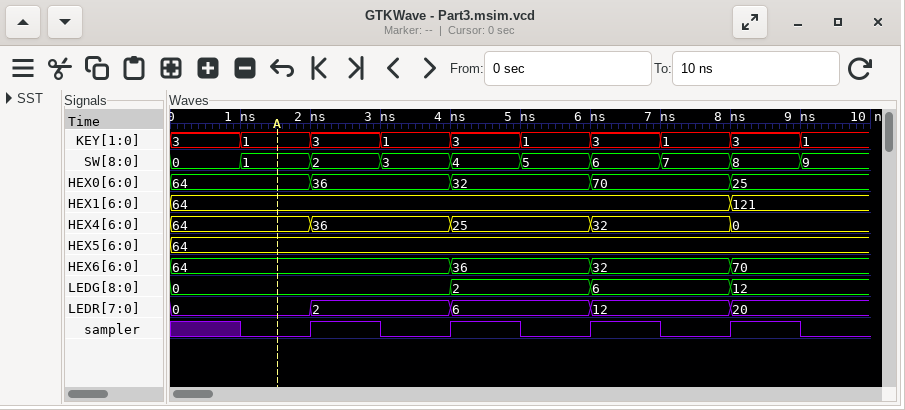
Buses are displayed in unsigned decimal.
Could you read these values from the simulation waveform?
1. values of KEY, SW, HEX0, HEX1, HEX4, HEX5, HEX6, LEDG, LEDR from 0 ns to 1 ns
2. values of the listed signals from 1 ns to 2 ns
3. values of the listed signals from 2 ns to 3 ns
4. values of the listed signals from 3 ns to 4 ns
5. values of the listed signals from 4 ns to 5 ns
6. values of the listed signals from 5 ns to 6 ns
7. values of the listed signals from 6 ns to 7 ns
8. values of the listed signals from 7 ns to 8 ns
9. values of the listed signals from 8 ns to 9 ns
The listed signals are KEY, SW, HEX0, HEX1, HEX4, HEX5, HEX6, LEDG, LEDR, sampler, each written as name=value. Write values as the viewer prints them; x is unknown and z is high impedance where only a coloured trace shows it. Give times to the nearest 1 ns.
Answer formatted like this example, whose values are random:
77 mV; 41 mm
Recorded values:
KEY=3, SW=0, HEX0=64, HEX1=64, HEX4=64, HEX5=64, HEX6=64, LEDG=0, LEDR=0; KEY=1, SW=1, HEX0=64, HEX1=64, HEX4=64, HEX5=64, HEX6=64, LEDG=0, LEDR=0, sampler=0; KEY=3, SW=2, HEX0=36, HEX1=64, HEX4=36, HEX5=64, HEX6=64, LEDG=0, LEDR=2, sampler=1; KEY=1, SW=3, HEX0=36, HEX1=64, HEX4=36, HEX5=64, HEX6=64, LEDG=0, LEDR=2, sampler=0; KEY=3, SW=4, HEX0=32, HEX1=64, HEX4=25, HEX5=64, HEX6=36, LEDG=2, LEDR=6, sampler=1; KEY=1, SW=5, HEX0=32, HEX1=64, HEX4=25, HEX5=64, HEX6=36, LEDG=2, LEDR=6, sampler=0; KEY=3, SW=6, HEX0=70, HEX1=64, HEX4=32, HEX5=64, HEX6=32, LEDG=6, LEDR=12, sampler=1; KEY=1, SW=7, HEX0=70, HEX1=64, HEX4=32, HEX5=64, HEX6=32, LEDG=6, LEDR=12, sampler=0; KEY=3, SW=8, HEX0=25, HEX1=121, HEX4=0, HEX5=64, HEX6=70, LEDG=12, LEDR=20, sampler=1
